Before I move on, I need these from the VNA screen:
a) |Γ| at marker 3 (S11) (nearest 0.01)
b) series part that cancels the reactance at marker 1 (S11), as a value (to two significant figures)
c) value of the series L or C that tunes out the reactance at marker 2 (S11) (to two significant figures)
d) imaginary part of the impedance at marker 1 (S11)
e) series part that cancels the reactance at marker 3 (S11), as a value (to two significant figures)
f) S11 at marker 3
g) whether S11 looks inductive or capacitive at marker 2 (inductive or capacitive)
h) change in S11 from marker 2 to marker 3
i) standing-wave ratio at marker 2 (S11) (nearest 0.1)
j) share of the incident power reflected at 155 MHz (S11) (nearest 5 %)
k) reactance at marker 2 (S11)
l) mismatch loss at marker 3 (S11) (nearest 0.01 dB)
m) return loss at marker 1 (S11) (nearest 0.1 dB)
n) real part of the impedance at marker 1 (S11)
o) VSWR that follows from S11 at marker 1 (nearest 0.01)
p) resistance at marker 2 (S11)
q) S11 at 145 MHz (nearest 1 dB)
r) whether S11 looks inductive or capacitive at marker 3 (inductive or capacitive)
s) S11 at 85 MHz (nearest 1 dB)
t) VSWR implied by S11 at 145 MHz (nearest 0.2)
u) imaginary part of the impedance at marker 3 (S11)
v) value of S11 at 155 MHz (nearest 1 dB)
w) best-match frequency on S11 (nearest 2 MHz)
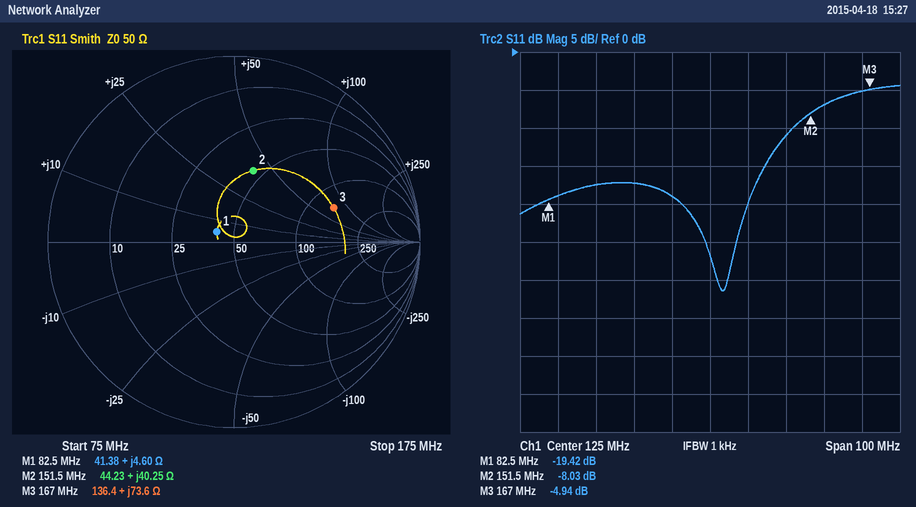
0.57
420 pF
26 pF
+4.60 Ω
13 pF
-4.94 dB
inductive
3.09 dB
2.3
20 %
+40.25 Ω
1.68 dB
19.4 dB
41.38 Ω
1.24
44.23 Ω
-11 dB
inductive
-19 dB
1.8
+73.6 Ω
-7 dB
128 MHz
